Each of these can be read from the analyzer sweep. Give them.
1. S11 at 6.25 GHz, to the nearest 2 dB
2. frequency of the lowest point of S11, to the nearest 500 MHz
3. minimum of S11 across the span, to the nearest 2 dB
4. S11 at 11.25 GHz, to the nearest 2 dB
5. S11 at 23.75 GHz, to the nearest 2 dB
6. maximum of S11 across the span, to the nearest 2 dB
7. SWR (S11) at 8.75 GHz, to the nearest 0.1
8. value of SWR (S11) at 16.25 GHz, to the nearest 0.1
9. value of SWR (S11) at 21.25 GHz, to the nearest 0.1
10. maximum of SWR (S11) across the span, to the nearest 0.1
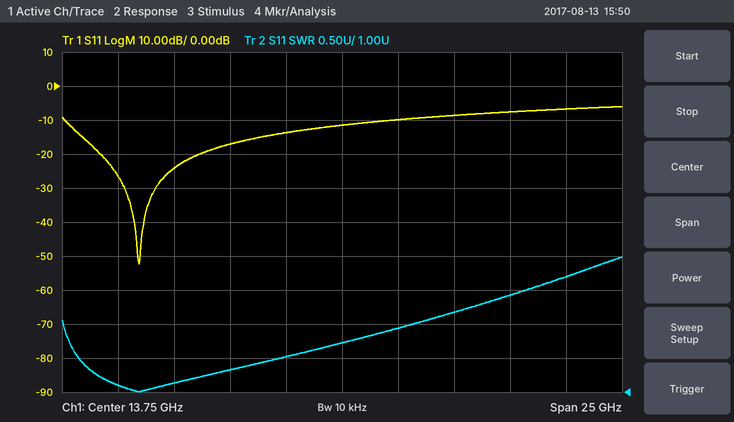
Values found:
-24 dB
4.5 GHz
-52 dB
-14 dB
-6 dB
-6 dB
1.3
1.9
2.4
3.0
